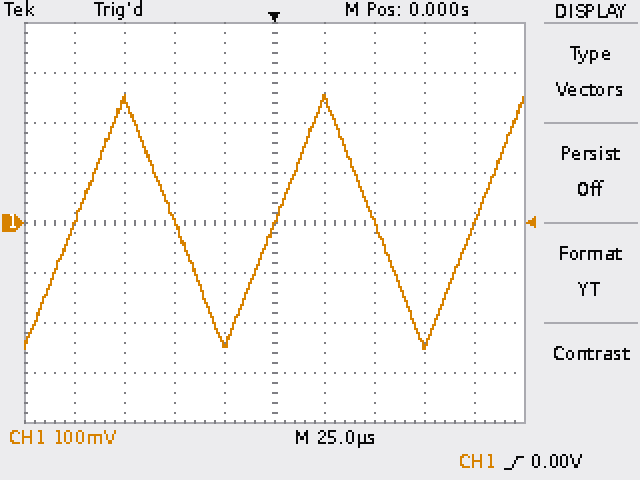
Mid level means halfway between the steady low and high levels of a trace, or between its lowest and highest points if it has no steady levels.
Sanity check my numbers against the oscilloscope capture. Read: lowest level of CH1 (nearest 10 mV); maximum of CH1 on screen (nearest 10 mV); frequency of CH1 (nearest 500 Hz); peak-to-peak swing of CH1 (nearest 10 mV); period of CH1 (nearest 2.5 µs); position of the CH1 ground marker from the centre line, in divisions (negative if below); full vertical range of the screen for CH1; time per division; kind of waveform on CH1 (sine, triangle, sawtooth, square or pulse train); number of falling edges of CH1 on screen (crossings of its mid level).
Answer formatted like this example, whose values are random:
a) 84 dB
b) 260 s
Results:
a) -250 mV
b) 260 mV
c) 10.0 kHz
d) 510 mV
e) 100.0 µs
f) 0.0 div
g) 800 mV
h) 25 µs
i) triangle
j) 2
